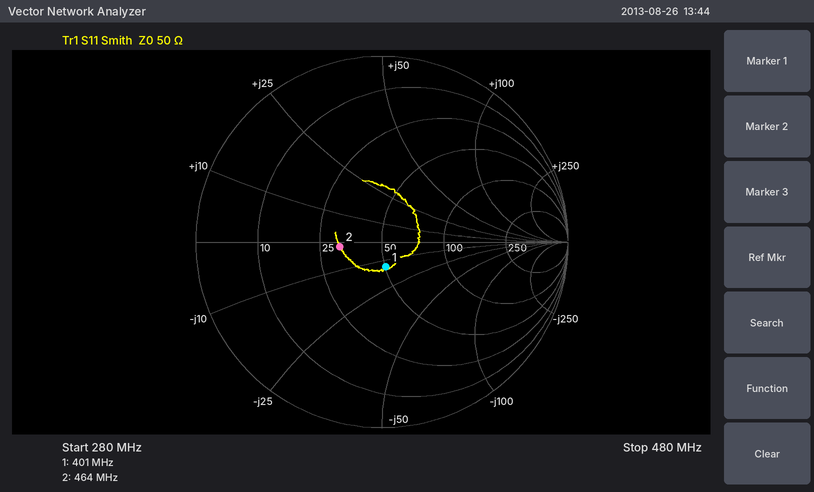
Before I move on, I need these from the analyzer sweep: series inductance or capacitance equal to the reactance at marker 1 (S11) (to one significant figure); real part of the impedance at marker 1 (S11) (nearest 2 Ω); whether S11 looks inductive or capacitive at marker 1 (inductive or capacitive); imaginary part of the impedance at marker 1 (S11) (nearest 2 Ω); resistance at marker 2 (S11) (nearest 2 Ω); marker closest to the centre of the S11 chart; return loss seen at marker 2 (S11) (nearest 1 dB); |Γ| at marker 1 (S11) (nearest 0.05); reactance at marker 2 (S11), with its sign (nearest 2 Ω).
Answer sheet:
30 pF
50 Ω
capacitive
-14 Ω
32 Ω
marker 1
13 dB
0.15
-2 Ω
